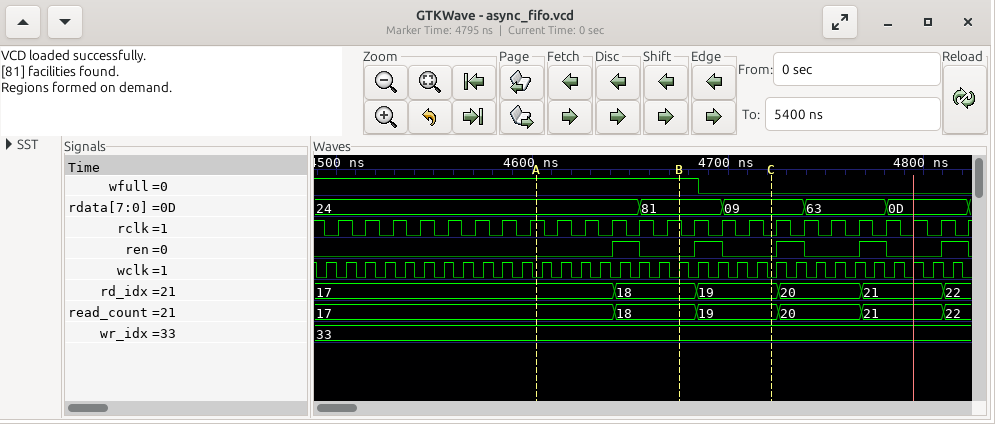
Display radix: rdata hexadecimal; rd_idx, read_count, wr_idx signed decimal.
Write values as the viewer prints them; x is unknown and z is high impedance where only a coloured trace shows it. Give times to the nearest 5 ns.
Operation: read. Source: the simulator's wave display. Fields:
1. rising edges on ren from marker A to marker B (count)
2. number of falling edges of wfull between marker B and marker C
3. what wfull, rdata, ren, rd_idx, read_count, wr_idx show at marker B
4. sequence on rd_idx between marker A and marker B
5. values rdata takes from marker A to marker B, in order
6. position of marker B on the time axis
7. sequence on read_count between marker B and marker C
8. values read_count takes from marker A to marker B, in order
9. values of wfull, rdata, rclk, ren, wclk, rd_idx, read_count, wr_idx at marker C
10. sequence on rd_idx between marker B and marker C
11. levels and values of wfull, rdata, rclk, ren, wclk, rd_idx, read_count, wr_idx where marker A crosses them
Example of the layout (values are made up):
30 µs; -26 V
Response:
1; 1; wfull=1, rdata=81, ren=0, rd_idx=18, read_count=18, wr_idx=33; 17, 18; 24, 81; 4675 ns; 18, 19; 17, 18; wfull=0, rdata=09, rclk=0, ren=0, wclk=0, rd_idx=19, read_count=19, wr_idx=33; 18, 19; wfull=1, rdata=24, rclk=1, ren=0, wclk=0, rd_idx=17, read_count=17, wr_idx=33
